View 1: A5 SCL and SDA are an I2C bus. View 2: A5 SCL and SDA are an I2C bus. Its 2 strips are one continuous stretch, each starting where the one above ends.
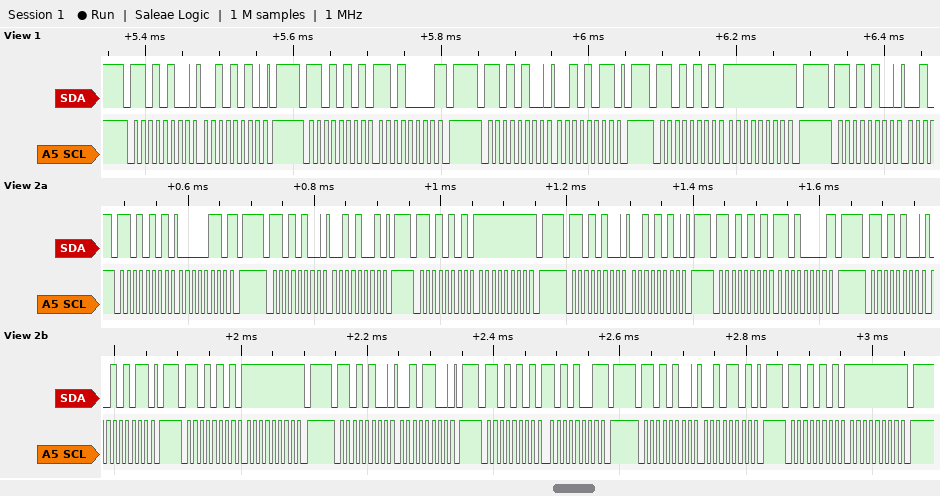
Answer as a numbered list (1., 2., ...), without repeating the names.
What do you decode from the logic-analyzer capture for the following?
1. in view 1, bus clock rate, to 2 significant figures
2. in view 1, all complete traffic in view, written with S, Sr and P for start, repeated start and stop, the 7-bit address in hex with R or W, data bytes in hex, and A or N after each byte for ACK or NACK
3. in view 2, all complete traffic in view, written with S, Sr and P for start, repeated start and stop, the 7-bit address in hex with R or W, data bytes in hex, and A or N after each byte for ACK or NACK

1. 100 kHz
2. S 6AW A 2A A P S 6AR A D0 N P S 6AW A 2B A P S 6AR A FF N P S 6AW A
3. S 6AR A 06 N P S 6AW A 29 A P S 6AR A FF N P S 6AW A 2A A P S 6AR A D0 N P S 6AW A 2B A P S 6AR A FF N P S 6AW A 2C A P S 6AR A A9 N P S 6AW A 2D A P S 6AR A FF N P
